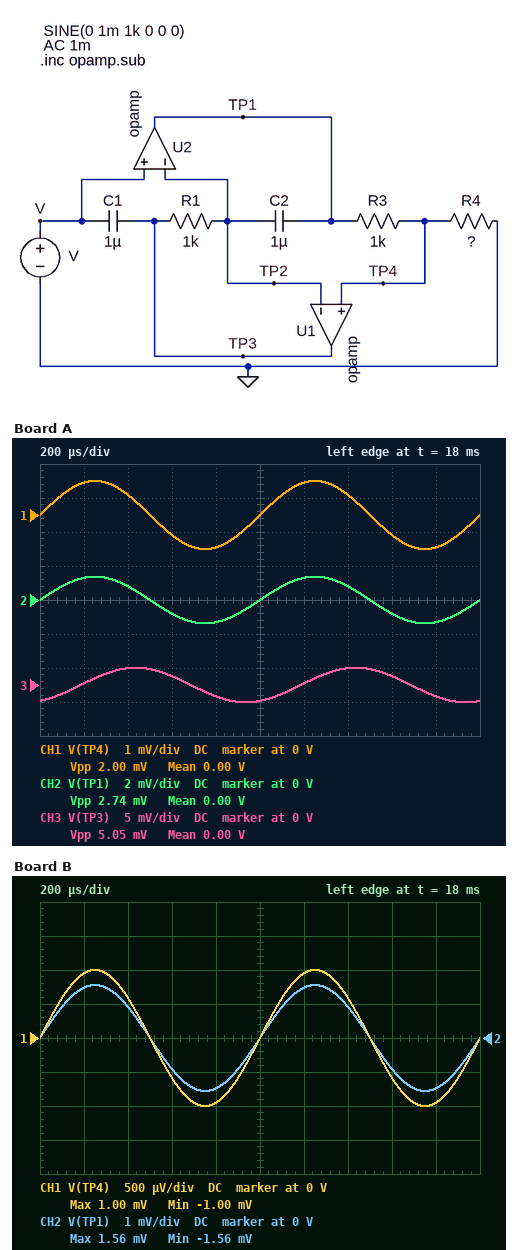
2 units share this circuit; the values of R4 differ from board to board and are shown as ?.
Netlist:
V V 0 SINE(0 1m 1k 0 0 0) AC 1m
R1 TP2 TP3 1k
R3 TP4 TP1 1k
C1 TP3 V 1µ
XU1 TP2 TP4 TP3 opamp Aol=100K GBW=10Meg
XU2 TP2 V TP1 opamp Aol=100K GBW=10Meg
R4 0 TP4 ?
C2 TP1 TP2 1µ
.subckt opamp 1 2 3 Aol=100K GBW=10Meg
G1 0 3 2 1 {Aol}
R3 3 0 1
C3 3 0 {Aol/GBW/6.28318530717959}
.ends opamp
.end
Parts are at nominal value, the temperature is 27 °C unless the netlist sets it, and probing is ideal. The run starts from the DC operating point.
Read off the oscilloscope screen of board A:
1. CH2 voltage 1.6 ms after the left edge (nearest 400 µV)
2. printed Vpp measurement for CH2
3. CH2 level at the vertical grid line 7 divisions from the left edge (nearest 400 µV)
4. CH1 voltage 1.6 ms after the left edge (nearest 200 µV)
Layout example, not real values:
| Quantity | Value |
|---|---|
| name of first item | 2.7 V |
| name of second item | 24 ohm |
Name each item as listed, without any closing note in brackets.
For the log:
| Quantity | Value |
|---|---|
| CH2 voltage 1.6 ms after the left edge | -800 µV |
| printed Vpp measurement for CH2 | 2.74 mV |
| CH2 level at the vertical grid line 7 divisions from the left edge | 800 µV |
| CH1 voltage 1.6 ms after the left edge | -600 µV |
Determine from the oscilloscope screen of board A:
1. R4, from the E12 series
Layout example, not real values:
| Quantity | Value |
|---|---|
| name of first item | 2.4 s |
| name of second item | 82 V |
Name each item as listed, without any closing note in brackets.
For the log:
| Quantity | Value |
|---|---|
| R4, from the E12 series | 2.7 kΩ |
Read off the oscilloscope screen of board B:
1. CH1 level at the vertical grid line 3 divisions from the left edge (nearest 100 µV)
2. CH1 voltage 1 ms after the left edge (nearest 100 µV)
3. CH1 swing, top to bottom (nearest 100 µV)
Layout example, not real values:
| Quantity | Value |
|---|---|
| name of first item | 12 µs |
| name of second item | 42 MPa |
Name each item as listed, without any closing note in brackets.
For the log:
| Quantity | Value |
|---|---|
| CH1 level at the vertical grid line 3 divisions from the left edge | -600 µV |
| CH1 voltage 1 ms after the left edge | 0 V |
| CH1 swing, top to bottom | 2.0 mV |
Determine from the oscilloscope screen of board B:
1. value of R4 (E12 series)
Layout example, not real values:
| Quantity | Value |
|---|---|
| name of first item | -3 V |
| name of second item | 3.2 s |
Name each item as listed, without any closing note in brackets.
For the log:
| Quantity | Value |
|---|---|
| value of R4 | 1.8 kΩ |
